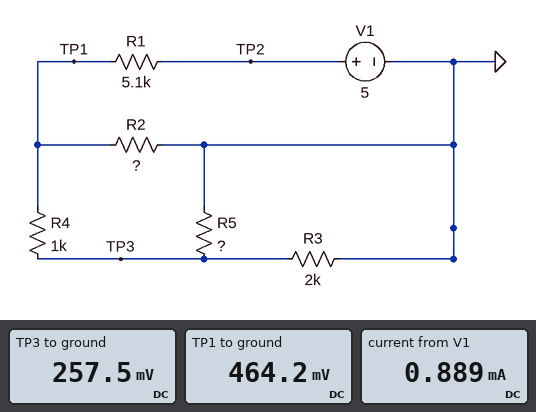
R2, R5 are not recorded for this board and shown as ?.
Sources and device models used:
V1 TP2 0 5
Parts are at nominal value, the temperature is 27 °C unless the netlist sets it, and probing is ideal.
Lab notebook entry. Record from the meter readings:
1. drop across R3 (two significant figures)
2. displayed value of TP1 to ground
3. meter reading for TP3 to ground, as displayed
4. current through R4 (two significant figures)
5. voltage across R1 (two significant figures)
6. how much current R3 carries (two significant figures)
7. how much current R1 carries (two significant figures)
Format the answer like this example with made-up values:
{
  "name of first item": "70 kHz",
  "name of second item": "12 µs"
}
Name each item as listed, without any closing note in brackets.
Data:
{
  "drop across R3": "260 mV",
  "displayed value of TP1 to ground": "464.2 mV",
  "meter reading for TP3 to ground, as displayed": "257.5 mV",
  "current through R4": "210 µA",
  "voltage across R1": "4.5 V",
  "how much current R3 carries": "130 µA",
  "how much current R1 carries": "890 µA"
}
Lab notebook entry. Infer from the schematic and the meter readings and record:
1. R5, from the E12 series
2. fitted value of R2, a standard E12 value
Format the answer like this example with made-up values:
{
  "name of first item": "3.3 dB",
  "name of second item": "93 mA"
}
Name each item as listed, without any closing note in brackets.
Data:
{
  "R5, from the E12 series": "3.3 kΩ",
  "fitted value of R2, a standard E12 value": "680 Ω"
}
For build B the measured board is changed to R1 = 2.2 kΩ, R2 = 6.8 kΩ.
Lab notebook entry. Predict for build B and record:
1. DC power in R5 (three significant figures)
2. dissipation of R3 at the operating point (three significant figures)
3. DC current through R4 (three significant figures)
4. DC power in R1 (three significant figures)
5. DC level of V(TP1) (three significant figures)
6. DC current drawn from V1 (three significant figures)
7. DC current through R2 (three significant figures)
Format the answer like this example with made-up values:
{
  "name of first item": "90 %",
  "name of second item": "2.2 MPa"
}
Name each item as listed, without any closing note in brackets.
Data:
{
  "DC power in R5": "439 µW",
  "dissipation of R3 at the operating point": "725 µW",
  "DC current through R4": "967 µA",
  "DC power in R1": "3.64 mW",
  "DC level of V(TP1)": "2.17 V",
  "DC current drawn from V1": "1.29 mA",
  "DC current through R2": "319 µA"
}
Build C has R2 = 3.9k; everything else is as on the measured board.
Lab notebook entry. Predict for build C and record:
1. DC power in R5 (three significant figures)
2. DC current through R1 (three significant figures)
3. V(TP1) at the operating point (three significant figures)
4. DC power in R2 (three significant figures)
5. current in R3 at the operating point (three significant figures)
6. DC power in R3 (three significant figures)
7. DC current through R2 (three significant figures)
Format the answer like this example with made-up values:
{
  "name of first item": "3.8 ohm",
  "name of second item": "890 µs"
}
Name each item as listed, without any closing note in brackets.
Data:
{
  "DC power in R5": "111 µW",
  "DC current through R1": "766 µA",
  "V(TP1) at the operating point": "1.09 V",
  "DC power in R2": "306 µW",
  "current in R3 at the operating point": "303 µA",
  "DC power in R3": "183 µW",
  "DC current through R2": "280 µA"
}
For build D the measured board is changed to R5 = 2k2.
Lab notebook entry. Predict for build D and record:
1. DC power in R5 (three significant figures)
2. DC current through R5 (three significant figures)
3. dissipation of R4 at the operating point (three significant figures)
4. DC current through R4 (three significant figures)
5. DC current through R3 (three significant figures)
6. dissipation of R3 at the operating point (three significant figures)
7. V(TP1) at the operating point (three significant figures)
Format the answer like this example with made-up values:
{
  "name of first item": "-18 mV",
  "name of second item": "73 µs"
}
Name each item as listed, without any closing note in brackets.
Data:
{
  "DC power in R5": "24.6 µW",
  "DC current through R5": "106 µA",
  "dissipation of R4 at the operating point": "49.4 µW",
  "DC current through R4": "222 µA",
  "DC current through R3": "116 µA",
  "dissipation of R3 at the operating point": "27.1 µW",
  "V(TP1) at the operating point": "455 mV"
}
